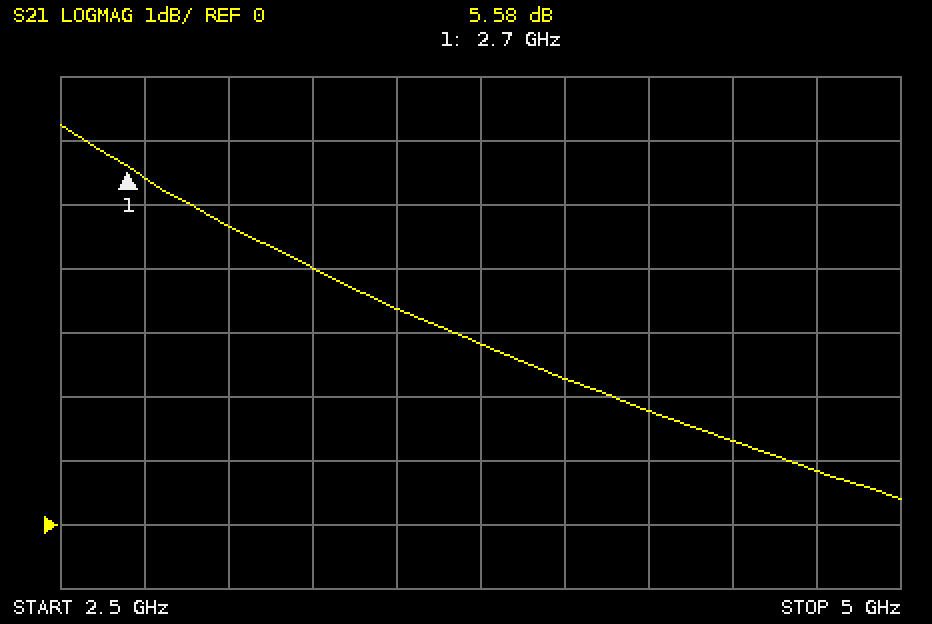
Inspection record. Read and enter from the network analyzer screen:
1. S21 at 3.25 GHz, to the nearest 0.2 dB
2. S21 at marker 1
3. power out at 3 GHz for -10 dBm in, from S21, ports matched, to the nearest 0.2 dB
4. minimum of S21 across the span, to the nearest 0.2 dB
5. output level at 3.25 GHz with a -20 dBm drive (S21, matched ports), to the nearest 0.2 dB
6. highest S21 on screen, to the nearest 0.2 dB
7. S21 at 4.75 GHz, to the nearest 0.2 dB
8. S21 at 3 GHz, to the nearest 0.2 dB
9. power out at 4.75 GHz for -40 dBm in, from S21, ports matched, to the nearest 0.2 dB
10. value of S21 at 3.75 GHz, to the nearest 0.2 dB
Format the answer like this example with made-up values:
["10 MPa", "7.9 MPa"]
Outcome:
["4.0 dB", "5.58 dB", "-5.4 dBm", "0.4 dB", "-16.0 dBm", "6.2 dB", "0.8 dB", "4.6 dB", "-39.2 dBm", "2.8 dB"]
